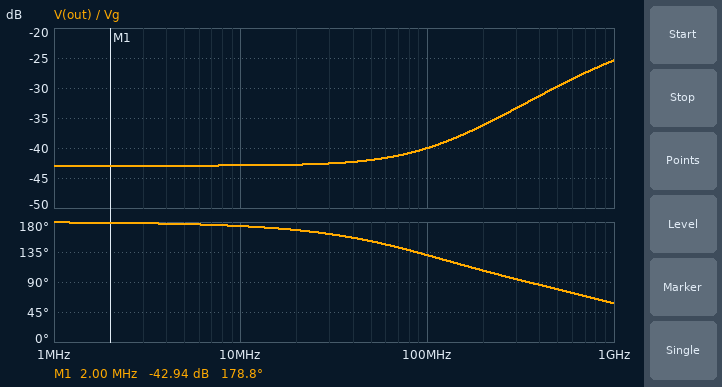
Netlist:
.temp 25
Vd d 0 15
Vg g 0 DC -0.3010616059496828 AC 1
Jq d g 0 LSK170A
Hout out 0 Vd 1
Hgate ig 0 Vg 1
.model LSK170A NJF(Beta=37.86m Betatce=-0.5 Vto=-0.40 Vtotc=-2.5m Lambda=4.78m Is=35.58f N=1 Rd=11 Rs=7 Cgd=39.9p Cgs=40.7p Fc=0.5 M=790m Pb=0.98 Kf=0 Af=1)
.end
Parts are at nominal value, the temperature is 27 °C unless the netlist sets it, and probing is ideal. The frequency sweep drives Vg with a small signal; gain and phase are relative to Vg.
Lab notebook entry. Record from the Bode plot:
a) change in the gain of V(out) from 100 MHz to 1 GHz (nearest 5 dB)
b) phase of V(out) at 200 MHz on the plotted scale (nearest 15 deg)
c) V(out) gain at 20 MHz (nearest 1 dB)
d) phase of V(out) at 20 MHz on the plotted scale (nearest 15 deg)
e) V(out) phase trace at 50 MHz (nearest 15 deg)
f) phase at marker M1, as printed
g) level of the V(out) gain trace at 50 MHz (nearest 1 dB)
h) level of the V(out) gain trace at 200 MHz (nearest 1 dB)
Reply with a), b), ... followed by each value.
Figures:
a) 15 dB
b) 105 deg
c) -43 dB
d) 165 deg
e) 150 deg
f) 178.8 deg
g) -42 dB
h) -36 dB
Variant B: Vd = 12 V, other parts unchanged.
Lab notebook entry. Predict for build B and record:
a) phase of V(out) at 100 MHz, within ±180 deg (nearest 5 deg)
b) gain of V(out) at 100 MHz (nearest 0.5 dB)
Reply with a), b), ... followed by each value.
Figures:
a) 125 deg
b) -39.5 dB
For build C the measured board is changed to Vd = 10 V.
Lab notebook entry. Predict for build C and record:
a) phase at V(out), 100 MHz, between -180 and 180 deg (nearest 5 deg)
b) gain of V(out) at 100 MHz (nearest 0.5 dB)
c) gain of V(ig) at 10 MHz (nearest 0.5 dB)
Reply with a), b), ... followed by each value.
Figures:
a) 125 deg
b) -39.5 dB
c) -50.5 dB
